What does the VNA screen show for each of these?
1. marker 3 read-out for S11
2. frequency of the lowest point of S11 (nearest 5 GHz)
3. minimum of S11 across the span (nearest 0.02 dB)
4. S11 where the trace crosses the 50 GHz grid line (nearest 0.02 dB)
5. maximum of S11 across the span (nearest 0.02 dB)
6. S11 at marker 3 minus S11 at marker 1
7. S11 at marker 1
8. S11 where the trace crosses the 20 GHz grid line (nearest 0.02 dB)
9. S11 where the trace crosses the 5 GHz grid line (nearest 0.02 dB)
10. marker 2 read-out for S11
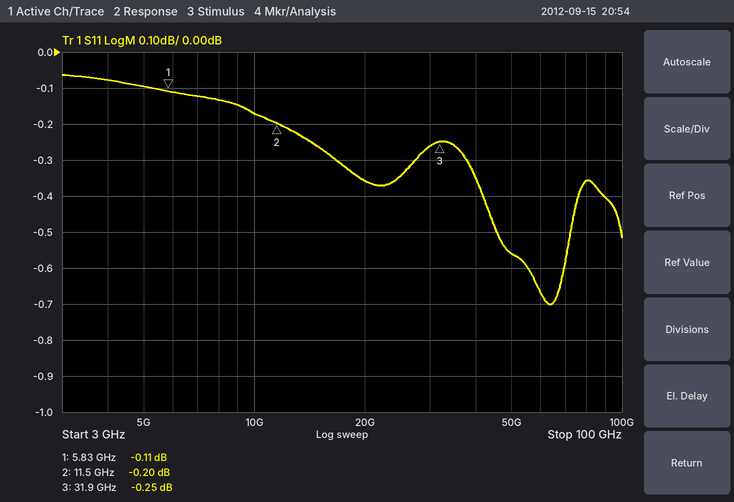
-0.25 dB
65 GHz
-0.70 dB
-0.56 dB
-0.06 dB
-0.14 dB
-0.11 dB
-0.36 dB
-0.10 dB
-0.20 dB
